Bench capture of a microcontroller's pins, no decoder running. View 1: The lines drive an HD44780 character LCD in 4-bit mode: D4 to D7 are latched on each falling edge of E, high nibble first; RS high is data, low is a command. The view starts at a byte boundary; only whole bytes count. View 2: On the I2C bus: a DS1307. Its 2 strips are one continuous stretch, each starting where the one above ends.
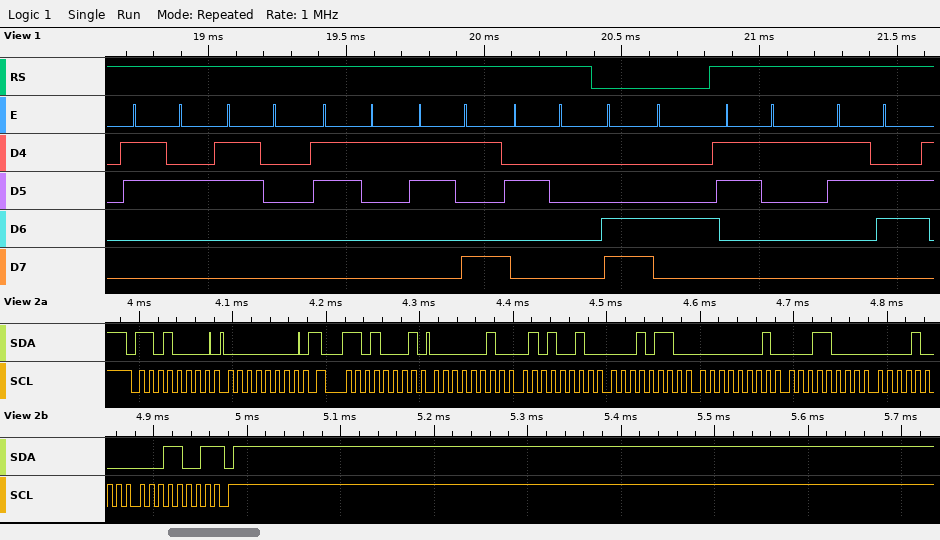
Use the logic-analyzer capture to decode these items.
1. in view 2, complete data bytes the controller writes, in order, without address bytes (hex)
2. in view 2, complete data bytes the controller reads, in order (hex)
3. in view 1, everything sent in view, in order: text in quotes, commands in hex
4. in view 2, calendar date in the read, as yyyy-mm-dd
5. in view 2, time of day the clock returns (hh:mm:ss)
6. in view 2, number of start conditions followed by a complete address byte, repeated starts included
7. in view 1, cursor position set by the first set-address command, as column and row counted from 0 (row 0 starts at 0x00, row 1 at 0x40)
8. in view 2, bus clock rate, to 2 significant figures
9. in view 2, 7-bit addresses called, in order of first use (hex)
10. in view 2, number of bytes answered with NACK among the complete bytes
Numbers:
00
02 52 16 01 18 08 19
"2019 " 0xC4 "16"
2019-08-18
16:52:02
2
column 4, row 1
100 kHz
0x68
1
